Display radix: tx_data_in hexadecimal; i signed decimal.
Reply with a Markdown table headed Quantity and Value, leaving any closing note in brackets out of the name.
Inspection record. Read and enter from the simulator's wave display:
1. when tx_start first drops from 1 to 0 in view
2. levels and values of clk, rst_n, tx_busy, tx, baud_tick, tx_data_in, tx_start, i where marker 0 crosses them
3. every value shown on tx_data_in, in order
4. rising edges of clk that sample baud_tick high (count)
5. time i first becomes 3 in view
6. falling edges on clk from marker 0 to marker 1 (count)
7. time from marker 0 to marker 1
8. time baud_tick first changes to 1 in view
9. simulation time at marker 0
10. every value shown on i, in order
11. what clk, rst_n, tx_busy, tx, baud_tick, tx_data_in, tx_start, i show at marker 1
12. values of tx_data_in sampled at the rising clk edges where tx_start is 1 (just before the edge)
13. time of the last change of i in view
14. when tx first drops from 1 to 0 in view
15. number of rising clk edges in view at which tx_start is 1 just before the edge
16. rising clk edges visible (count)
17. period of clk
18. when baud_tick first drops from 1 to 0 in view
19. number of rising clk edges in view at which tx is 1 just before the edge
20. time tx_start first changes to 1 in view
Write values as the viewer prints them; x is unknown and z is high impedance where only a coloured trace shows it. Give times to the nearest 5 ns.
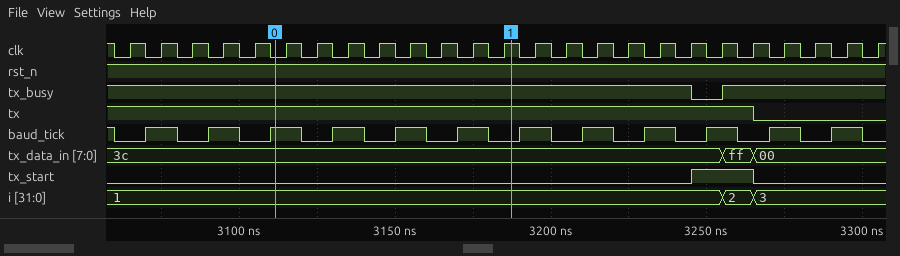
| Quantity | Value |
|---|---|
| when tx_start first drops from 1 to 0 in view | 3265 ns |
| levels and values of clk, rst_n, tx_busy, tx, baud_tick, tx_data_in, tx_start, i where marker 0 crosses them | clk=0, rst_n=1, tx_busy=1, tx=1, baud_tick=1, tx_data_in=3c, tx_start=0, i=1 |
| every value shown on tx_data_in, in order | 3c, ff, 00 |
| rising edges of clk that sample baud_tick high | 12 |
| time i first becomes 3 in view | 3265 ns |
| falling edges on clk from marker 0 to marker 1 | 7 |
| time from marker 0 to marker 1 | 75 ns |
| time baud_tick first changes to 1 in view | 3070 ns |
| simulation time at marker 0 | 3110 ns |
| every value shown on i, in order | 1, 2, 3 |
| what clk, rst_n, tx_busy, tx, baud_tick, tx_data_in, tx_start, i show at marker 1 | clk=1, rst_n=1, tx_busy=1, tx=1, baud_tick=0, tx_data_in=3c, tx_start=0, i=1 |
| values of tx_data_in sampled at the rising clk edges where tx_start is 1 | 3c, ff |
| time of the last change of i in view | 3265 ns |
| when tx first drops from 1 to 0 in view | 3265 ns |
| number of rising clk edges in view at which tx_start is 1 just before the edge | 2 |
| rising clk edges visible | 25 |
| period of clk | 10 ns |
| when baud_tick first drops from 1 to 0 in view | 3060 ns |
| number of rising clk edges in view at which tx is 1 just before the edge | 21 |
| time tx_start first changes to 1 in view | 3245 ns |
